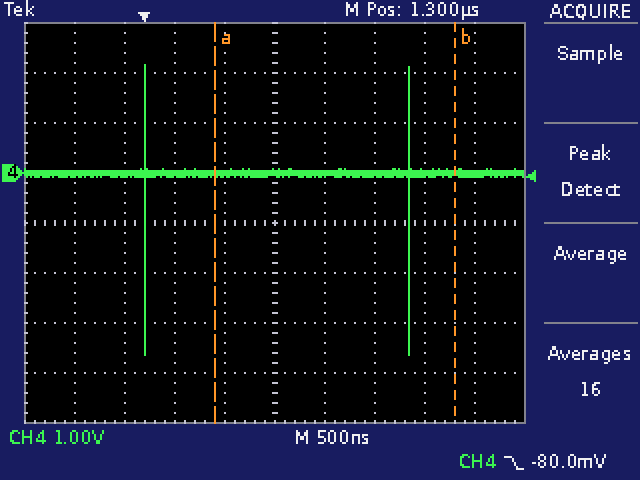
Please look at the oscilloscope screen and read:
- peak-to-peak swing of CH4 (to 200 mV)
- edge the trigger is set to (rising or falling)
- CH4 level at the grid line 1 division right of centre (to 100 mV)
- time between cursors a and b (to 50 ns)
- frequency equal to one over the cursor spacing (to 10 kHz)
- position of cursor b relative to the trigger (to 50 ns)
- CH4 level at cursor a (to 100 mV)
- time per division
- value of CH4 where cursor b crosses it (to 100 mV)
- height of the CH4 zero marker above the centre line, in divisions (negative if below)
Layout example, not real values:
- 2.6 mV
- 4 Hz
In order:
- 5.8 V
- falling
- 0.0 V
- 2.40 µs
- 420 kHz
- +3.10 µs
- 0.0 V
- 500 ns
- 0.0 V
- +1.0 div
